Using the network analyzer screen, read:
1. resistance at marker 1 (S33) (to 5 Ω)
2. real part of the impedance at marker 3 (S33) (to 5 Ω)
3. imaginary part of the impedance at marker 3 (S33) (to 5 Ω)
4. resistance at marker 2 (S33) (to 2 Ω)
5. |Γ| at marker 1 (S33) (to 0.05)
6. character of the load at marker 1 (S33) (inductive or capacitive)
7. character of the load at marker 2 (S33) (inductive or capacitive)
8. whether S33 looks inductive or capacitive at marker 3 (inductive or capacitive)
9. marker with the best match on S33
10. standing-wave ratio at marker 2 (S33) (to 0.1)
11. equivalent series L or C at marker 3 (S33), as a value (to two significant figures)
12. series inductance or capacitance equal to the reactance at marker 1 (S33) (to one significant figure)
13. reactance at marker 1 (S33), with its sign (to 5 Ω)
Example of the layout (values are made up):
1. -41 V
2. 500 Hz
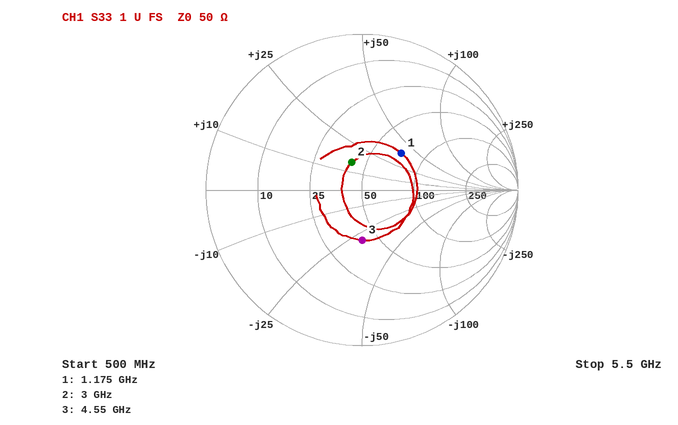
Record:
1. 70 Ω
2. 40 Ω
3. -30 Ω
4. 42 Ω
5. 0.35
6. inductive
7. inductive
8. capacitive
9. marker 2
10. 1.5
11. 1.2 pF
12. 5 nH
13. +40 Ω
